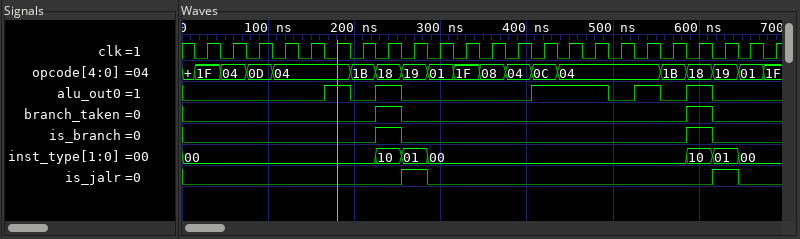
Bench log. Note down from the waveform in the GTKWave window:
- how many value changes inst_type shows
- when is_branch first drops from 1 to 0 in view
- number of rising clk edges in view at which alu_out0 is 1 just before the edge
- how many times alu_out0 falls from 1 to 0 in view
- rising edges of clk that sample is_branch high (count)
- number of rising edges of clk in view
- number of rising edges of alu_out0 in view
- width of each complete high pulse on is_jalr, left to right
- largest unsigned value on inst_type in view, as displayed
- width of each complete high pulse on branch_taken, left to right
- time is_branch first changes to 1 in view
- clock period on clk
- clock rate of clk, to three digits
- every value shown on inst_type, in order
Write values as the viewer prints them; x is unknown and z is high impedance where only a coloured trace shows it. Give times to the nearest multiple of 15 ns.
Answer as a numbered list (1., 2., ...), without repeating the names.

1. 6
2. 255 ns
3. 7
4. 5
5. 2
6. 23
7. 5
8. 30 ns, 30 ns
9. 10
10. 30 ns, 30 ns
11. 225 ns
12. 30 ns
13. 33.3 MHz
14. 00, 10, 01, 00, 10, 01, 00
